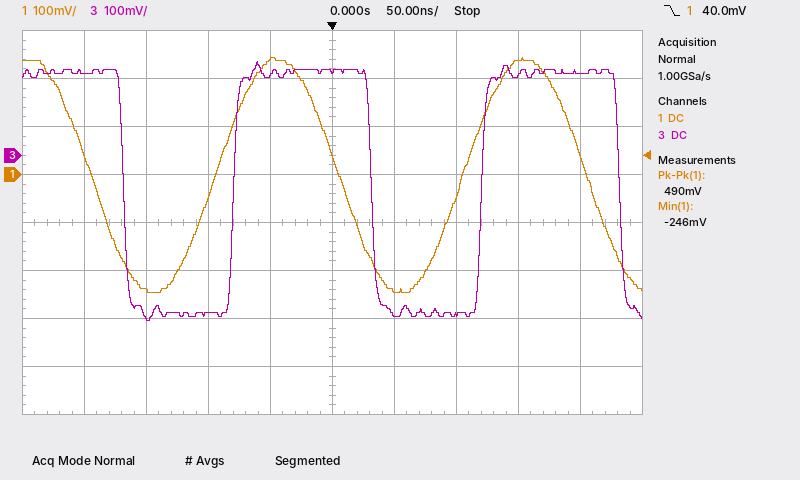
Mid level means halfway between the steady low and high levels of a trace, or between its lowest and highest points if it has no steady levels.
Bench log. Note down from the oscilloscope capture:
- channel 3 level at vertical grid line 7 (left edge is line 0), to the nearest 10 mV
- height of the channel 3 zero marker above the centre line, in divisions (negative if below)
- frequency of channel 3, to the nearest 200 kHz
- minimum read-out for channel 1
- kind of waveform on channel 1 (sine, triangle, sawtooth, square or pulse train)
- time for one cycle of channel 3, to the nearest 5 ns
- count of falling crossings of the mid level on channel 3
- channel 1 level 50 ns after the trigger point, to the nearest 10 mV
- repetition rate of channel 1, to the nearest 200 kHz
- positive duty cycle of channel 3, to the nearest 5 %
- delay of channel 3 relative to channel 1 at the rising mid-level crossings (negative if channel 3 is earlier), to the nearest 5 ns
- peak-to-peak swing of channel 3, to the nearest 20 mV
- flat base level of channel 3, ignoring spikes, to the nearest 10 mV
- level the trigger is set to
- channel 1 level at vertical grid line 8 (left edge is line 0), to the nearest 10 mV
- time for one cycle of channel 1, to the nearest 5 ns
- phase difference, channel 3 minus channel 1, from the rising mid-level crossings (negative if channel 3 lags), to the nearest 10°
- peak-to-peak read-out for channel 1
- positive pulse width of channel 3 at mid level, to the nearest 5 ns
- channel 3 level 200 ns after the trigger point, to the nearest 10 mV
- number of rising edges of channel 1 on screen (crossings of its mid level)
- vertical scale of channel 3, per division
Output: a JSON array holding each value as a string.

["-330 mV", "+1.4 div", "5.0 MHz", "-246 mV", "sine", "200 ns", "3", "-240 mV", "5.0 MHz", "55 %", "+15 ns", "540 mV", "-330 mV", "40.0 mV", "240 mV", "200 ns", "-30°", "490 mV", "110 ns", "170 mV", "2", "100 mV"]
